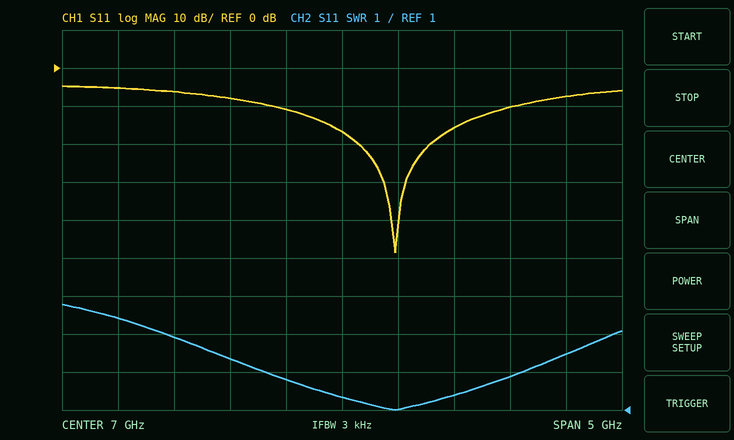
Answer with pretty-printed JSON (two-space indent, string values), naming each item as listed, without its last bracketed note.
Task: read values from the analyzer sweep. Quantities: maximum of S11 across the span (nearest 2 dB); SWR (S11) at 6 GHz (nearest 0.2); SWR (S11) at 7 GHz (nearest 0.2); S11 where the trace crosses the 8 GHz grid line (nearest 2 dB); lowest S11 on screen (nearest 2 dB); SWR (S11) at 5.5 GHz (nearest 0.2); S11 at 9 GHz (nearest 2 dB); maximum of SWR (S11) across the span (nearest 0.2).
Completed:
{
  "maximum of S11 across the span": "-4 dB",
  "SWR (S11) at 6 GHz": "2.4",
  "SWR (S11) at 7 GHz": "1.4",
  "S11 where the trace crosses the 8 GHz grid line": "-16 dB",
  "lowest S11 on screen": "-48 dB",
  "SWR (S11) at 5.5 GHz": "3.0",
  "S11 at 9 GHz": "-8 dB",
  "maximum of SWR (S11) across the span": "3.8"
}
